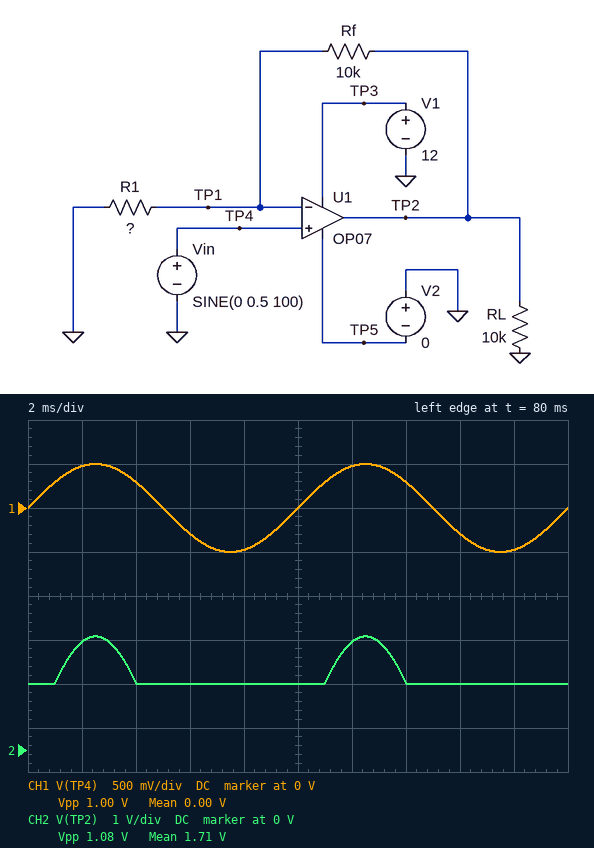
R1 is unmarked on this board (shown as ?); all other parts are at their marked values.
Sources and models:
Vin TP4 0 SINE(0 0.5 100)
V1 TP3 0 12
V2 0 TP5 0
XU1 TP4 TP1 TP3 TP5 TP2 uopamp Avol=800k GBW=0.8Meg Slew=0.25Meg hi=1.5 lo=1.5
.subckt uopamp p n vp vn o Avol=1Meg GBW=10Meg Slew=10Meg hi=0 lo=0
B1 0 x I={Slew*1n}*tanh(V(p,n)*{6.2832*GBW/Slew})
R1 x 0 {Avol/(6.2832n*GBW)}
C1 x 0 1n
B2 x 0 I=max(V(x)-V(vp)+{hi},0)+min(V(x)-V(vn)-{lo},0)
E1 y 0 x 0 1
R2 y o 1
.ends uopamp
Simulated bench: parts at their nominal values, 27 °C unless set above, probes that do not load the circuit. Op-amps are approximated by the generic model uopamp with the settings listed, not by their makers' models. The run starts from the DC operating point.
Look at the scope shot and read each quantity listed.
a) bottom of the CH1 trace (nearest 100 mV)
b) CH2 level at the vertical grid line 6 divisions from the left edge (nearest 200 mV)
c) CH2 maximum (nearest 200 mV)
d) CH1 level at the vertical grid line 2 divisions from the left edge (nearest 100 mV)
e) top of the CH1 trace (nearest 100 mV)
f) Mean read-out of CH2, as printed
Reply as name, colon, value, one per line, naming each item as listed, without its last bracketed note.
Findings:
bottom of the CH1 trace: -500 mV
CH2 level at the vertical grid line 6 divisions from the left edge: 2.4 V
CH2 maximum: 2.6 V
CH1 level at the vertical grid line 2 divisions from the left edge: 300 mV
top of the CH1 trace: 500 mV
Mean read-out of CH2, as printed: 1.71 V
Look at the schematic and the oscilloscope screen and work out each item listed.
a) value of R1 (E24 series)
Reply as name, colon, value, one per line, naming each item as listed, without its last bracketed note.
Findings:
value of R1: 2.4 kΩ
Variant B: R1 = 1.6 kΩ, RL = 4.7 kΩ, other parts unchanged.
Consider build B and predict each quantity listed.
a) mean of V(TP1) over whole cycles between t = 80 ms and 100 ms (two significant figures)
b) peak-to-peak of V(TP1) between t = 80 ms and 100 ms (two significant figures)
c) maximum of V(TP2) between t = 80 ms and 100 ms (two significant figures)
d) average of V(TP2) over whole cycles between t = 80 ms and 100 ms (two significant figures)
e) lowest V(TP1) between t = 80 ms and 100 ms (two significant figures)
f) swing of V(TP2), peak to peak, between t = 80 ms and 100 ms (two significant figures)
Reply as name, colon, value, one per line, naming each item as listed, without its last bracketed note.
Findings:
mean of V(TP1) over whole cycles between t = 80 ms and 100 ms: 280 mV
peak-to-peak of V(TP1) between t = 80 ms and 100 ms: 290 mV
maximum of V(TP2) between t = 80 ms and 100 ms: 3.6 V
average of V(TP2) over whole cycles between t = 80 ms and 100 ms: 2.0 V
lowest V(TP1) between t = 80 ms and 100 ms: 210 mV
swing of V(TP2), peak to peak, between t = 80 ms and 100 ms: 2.1 V
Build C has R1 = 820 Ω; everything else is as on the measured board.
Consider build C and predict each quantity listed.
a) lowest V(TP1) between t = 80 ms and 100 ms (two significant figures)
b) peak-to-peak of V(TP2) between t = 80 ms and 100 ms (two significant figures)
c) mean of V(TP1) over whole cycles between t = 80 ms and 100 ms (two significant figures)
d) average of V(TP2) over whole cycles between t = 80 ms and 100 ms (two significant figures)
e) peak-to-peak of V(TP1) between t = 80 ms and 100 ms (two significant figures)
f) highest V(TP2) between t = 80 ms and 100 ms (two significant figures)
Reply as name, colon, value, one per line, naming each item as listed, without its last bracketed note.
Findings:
lowest V(TP1) between t = 80 ms and 100 ms: 110 mV
peak-to-peak of V(TP2) between t = 80 ms and 100 ms: 5.1 V
mean of V(TP1) over whole cycles between t = 80 ms and 100 ms: 220 mV
average of V(TP2) over whole cycles between t = 80 ms and 100 ms: 2.9 V
peak-to-peak of V(TP1) between t = 80 ms and 100 ms: 390 mV
highest V(TP2) between t = 80 ms and 100 ms: 6.6 V
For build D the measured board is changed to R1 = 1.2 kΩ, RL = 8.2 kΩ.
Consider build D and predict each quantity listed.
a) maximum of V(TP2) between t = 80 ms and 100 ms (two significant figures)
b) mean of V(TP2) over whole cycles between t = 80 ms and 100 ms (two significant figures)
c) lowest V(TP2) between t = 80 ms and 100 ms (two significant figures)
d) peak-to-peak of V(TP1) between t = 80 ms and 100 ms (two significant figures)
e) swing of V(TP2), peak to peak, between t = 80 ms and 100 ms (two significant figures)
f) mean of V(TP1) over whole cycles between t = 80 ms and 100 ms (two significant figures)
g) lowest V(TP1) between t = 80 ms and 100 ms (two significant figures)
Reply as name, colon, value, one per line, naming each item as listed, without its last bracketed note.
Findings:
maximum of V(TP2) between t = 80 ms and 100 ms: 4.7 V
mean of V(TP2) over whole cycles between t = 80 ms and 100 ms: 2.3 V
lowest V(TP2) between t = 80 ms and 100 ms: 1.5 V
peak-to-peak of V(TP1) between t = 80 ms and 100 ms: 340 mV
swing of V(TP2), peak to peak, between t = 80 ms and 100 ms: 3.2 V
mean of V(TP1) over whole cycles between t = 80 ms and 100 ms: 250 mV
lowest V(TP1) between t = 80 ms and 100 ms: 160 mV
